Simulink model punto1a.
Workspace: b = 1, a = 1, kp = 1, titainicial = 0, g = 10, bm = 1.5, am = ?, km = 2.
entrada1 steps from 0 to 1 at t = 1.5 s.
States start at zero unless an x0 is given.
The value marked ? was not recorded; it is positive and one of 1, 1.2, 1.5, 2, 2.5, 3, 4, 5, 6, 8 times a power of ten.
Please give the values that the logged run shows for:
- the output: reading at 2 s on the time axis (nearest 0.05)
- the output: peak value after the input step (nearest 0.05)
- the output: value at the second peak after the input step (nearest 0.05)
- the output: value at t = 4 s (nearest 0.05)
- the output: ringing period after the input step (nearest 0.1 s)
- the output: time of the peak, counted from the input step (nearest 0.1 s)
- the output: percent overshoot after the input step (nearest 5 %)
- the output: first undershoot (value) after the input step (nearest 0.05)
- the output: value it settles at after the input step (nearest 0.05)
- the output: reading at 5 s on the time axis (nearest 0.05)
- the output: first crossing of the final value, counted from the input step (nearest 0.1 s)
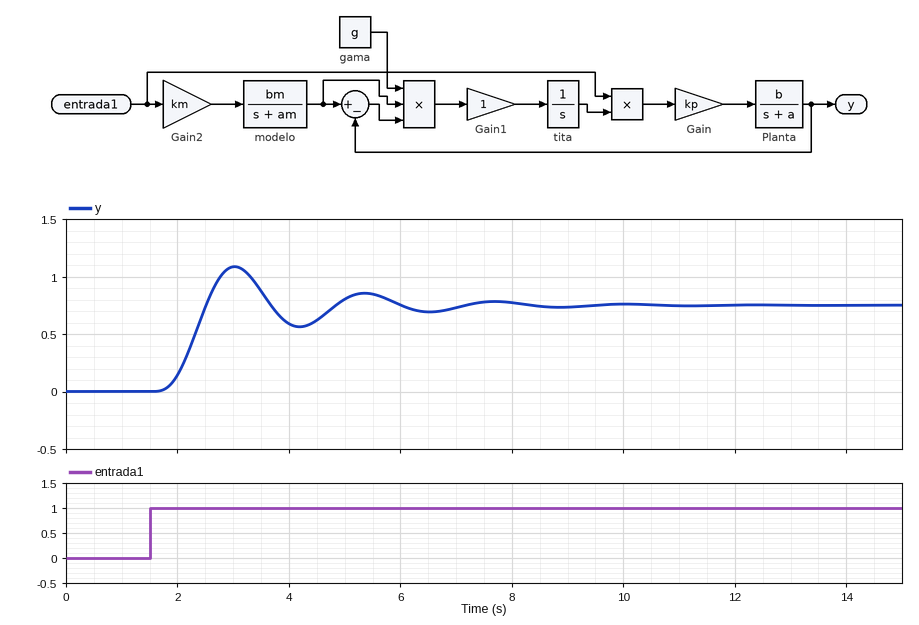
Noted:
0.15
1.10
0.85
0.60
2.3 s
1.5 s
45 %
0.55
0.75
0.80
1.0 s
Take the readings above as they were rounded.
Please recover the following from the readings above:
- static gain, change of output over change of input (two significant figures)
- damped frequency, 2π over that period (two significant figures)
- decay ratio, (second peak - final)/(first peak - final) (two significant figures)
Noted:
0.75
2.7 rad/s
0.29
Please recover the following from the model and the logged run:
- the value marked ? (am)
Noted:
4
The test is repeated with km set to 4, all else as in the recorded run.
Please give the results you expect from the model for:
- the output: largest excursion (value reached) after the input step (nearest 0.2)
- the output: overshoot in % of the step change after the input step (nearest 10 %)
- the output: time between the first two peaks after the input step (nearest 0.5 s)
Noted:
2.2
50 %
1.5 s
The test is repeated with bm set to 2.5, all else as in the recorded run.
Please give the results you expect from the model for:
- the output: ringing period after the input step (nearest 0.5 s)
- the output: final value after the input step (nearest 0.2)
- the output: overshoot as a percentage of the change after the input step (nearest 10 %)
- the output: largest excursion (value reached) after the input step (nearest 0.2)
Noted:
2.0 s
1.2
50 %
1.8
